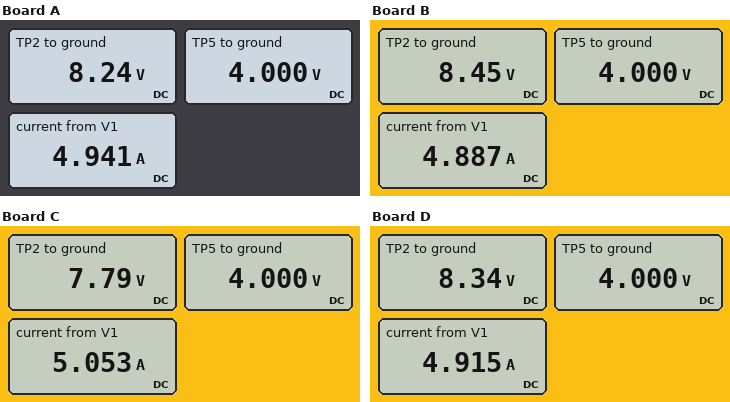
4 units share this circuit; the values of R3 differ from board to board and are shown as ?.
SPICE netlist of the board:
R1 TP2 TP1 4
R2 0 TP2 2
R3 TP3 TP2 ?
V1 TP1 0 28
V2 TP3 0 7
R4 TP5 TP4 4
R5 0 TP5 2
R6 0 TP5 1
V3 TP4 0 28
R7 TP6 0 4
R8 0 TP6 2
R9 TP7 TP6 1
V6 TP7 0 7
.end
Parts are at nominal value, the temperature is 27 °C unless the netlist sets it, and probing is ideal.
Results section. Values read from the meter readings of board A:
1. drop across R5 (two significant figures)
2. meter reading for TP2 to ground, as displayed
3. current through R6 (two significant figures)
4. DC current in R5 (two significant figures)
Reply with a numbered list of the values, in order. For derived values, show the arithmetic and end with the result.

1. 4 V = 4.0 V
2. 8.24 V
3. (4 V) / 1 Ω = 4.0 A
4. (4 V) / 2 Ω = 2.0 A
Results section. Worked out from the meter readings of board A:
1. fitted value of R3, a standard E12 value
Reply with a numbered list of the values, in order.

1. 1.5 Ω
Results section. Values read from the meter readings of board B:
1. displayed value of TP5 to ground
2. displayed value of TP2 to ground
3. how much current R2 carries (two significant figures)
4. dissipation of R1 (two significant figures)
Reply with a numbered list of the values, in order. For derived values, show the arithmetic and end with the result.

1. 4.000 V
2. 8.45 V
3. (8.45 V) / 2 Ω = 4.2 A
4. (28 V - 8.45 V)^2 / 4 Ω = 96 W
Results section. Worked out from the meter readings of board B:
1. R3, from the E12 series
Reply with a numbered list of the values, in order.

1. 2.2 Ω
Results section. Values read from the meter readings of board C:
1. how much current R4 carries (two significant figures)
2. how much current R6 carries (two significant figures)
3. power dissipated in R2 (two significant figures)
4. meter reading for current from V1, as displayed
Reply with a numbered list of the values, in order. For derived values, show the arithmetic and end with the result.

1. (28 V - 4 V) / 4 Ω = 6.0 A
2. (4 V) / 1 Ω = 4.0 A
3. (7.79 V)^2 / 2 Ω = 30 W
4. 5.053 A
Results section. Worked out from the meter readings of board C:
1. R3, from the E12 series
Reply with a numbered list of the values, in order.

1. 0.68 Ω
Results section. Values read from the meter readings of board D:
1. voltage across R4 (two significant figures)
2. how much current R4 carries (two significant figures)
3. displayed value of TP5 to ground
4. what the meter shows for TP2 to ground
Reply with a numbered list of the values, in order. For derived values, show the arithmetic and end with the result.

1. 28 V - 4 V = 24 V
2. (28 V - 4 V) / 4 Ω = 6.0 A
3. 4.000 V
4. 8.34 V
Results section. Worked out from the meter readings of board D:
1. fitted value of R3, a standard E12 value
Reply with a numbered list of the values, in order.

1. 1.8 Ω
